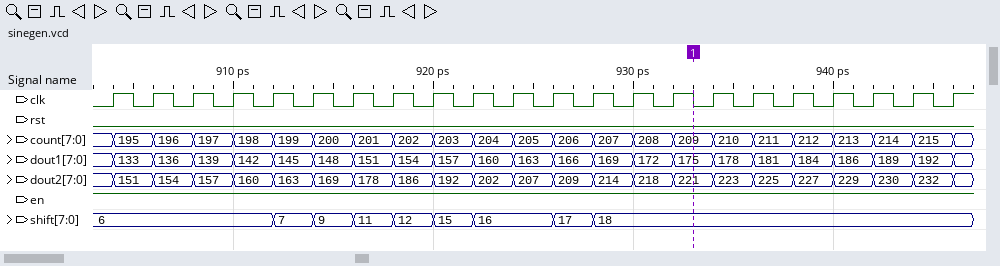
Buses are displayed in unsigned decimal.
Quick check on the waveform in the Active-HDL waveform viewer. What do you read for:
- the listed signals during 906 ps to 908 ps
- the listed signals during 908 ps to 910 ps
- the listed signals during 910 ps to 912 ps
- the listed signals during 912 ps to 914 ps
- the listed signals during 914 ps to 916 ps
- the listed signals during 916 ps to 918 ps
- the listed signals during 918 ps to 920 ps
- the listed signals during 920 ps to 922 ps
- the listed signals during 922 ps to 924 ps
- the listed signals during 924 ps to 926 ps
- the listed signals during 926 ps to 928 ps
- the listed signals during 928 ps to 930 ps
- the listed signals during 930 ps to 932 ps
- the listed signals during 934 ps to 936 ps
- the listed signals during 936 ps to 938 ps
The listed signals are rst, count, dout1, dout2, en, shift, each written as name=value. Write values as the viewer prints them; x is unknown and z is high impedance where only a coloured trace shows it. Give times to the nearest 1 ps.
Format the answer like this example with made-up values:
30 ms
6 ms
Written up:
rst=0, count=196, dout1=136, dout2=154, en=1, shift=6
rst=0, count=197, dout1=139, dout2=157, en=1, shift=6
rst=0, count=198, dout1=142, dout2=160, en=1, shift=6
rst=0, count=199, dout1=145, dout2=163, en=1, shift=7
rst=0, count=200, dout1=148, dout2=169, en=1, shift=9
rst=0, count=201, dout1=151, dout2=178, en=1, shift=11
rst=0, count=202, dout1=154, dout2=186, en=1, shift=12
rst=0, count=203, dout1=157, dout2=192, en=1, shift=15
rst=0, count=204, dout1=160, dout2=202, en=1, shift=16
rst=0, count=205, dout1=163, dout2=207, en=1, shift=16
rst=0, count=206, dout1=166, dout2=209, en=1, shift=17
rst=0, count=207, dout1=169, dout2=214, en=1, shift=18
rst=0, count=208, dout1=172, dout2=218, en=1, shift=18
rst=0, count=210, dout1=178, dout2=223, en=1, shift=18
rst=0, count=211, dout1=181, dout2=225, en=1, shift=18
